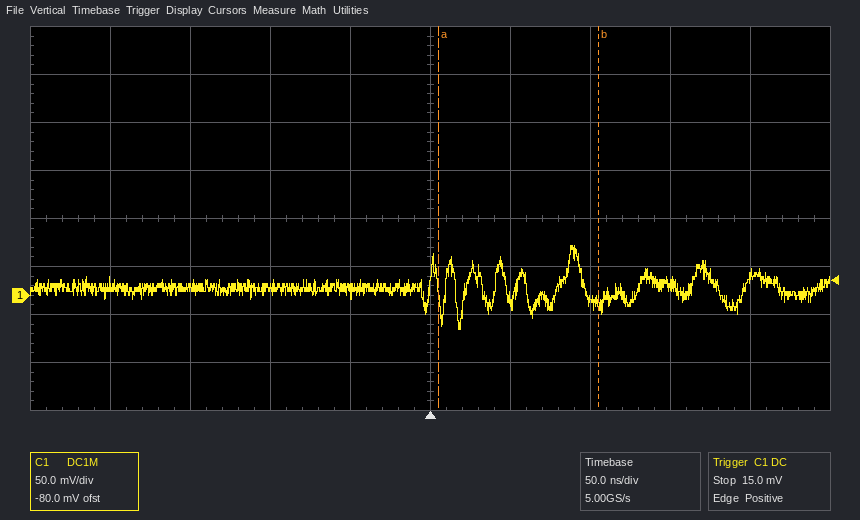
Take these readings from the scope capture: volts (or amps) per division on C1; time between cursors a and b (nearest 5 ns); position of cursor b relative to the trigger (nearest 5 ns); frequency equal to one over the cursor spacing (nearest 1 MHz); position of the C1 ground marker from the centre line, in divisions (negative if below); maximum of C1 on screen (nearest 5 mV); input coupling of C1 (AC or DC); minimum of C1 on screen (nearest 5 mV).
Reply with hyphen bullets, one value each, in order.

- 50 mV
- 100 ns
- +105 ns
- 10 MHz
- -1.6 div
- 50 mV
- DC
- -35 mV
